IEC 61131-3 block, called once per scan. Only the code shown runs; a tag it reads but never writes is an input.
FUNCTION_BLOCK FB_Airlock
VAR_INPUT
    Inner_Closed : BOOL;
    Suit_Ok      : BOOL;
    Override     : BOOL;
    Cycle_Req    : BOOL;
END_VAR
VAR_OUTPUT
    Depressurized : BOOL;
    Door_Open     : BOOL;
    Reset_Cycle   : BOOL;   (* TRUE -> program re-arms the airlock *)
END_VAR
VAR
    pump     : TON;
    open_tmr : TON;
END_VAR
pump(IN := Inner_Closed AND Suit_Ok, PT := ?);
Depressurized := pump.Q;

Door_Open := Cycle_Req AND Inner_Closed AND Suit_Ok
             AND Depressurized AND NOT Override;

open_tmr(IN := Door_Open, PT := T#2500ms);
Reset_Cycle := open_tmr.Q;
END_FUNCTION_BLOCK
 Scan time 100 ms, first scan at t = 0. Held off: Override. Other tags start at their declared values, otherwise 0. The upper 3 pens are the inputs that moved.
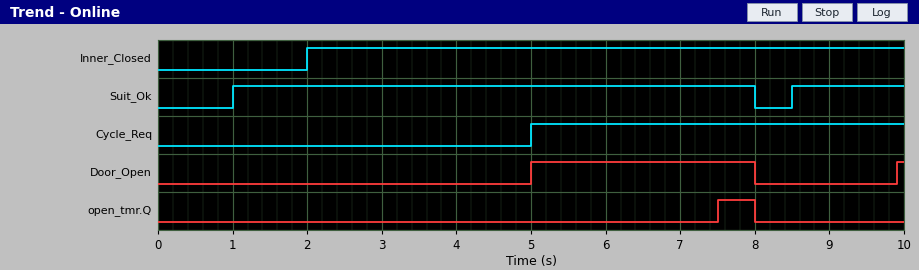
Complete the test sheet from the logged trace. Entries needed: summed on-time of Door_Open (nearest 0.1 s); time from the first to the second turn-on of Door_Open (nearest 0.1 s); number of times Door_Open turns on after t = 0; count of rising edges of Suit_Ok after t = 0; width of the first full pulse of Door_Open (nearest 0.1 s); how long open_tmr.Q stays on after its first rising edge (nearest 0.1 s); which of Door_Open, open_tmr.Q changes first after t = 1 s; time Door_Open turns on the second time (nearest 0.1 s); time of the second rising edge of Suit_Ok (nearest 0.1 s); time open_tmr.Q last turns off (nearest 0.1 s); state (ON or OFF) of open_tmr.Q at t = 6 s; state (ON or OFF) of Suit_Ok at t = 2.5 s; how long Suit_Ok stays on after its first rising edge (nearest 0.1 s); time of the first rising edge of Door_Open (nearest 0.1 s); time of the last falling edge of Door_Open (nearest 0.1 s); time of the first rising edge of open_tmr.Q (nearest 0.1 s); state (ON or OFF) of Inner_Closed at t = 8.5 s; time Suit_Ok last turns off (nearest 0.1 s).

3.1 s
4.9 s
2
2
3.0 s
0.5 s
Door_Open
9.9 s
8.5 s
8.0 s
OFF
ON
7.0 s
5.0 s
8.0 s
7.5 s
ON
8.0 s
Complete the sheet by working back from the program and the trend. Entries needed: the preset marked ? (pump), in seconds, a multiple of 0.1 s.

1.4 s
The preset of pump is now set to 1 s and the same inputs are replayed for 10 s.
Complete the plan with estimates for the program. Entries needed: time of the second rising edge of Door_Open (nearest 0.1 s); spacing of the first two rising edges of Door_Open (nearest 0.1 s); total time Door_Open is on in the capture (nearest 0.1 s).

9.5 s
4.5 s
3.5 s
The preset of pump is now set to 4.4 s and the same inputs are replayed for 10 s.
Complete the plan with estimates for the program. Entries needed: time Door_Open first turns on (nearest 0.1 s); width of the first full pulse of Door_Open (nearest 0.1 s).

6.4 s
1.6 s
